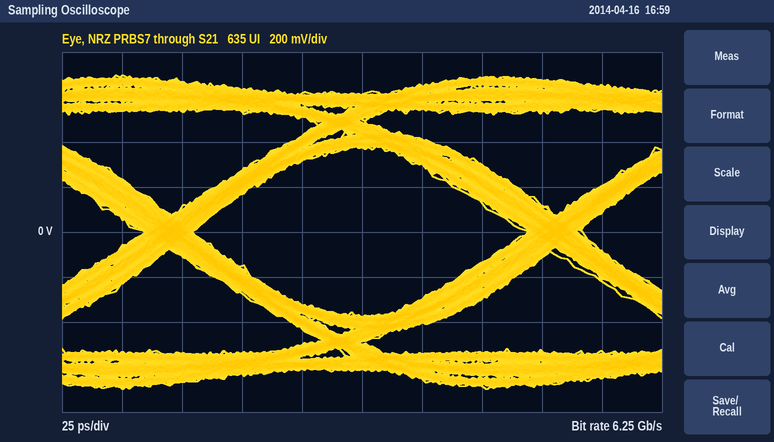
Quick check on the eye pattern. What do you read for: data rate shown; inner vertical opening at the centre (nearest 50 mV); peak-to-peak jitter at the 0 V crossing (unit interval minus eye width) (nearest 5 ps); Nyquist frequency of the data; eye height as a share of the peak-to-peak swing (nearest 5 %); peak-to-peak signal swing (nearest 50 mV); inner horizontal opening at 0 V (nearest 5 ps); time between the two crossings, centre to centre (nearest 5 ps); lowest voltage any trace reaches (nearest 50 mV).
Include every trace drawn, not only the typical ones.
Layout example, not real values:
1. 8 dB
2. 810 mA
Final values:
1. 6.25 Gb/s
2. 750 mV
3. 20 ps
4. 3.125 GHz
5. 55 %
6. 1.40 V
7. 140 ps
8. 160 ps
9. -700 mV
